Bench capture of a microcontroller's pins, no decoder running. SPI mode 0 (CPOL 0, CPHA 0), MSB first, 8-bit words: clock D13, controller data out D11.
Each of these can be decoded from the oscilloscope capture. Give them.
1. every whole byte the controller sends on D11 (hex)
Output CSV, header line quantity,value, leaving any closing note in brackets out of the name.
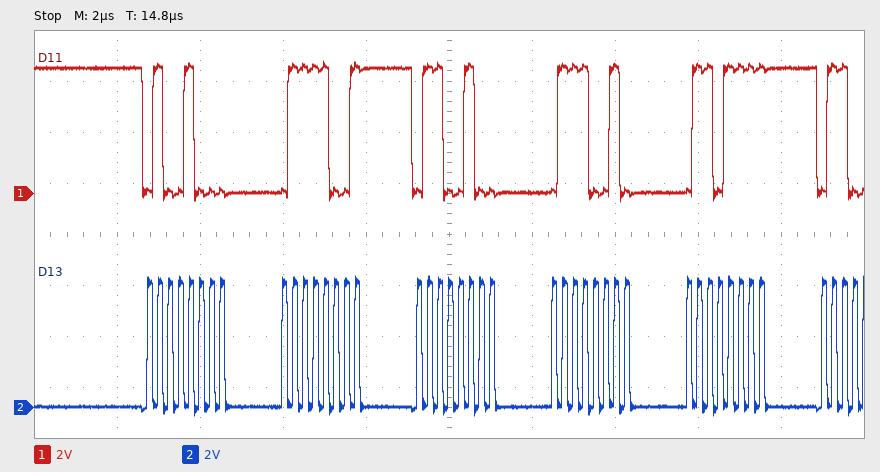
quantity,value
every whole byte the controller sends on D11,48 79 64 72 6F
